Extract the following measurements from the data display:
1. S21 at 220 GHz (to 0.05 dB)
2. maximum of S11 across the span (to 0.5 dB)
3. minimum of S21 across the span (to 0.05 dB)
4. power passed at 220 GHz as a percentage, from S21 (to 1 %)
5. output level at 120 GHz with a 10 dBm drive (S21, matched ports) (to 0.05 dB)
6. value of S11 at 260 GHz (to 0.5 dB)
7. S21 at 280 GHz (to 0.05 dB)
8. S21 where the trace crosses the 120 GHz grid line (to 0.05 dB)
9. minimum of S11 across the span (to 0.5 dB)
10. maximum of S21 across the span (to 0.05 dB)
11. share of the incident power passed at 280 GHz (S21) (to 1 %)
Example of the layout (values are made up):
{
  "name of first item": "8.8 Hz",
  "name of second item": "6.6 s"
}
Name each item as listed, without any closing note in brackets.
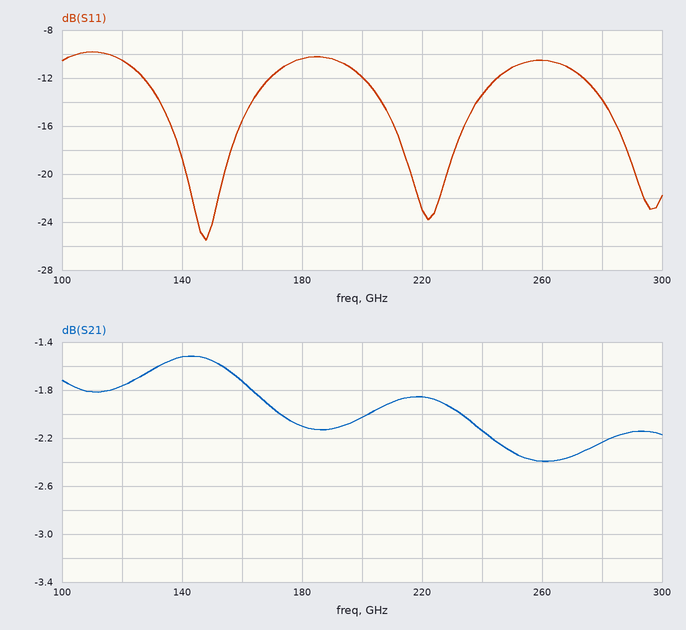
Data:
{
  "S21 at 220 GHz": "-1.85 dB",
  "maximum of S11 across the span": "-10.0 dB",
  "minimum of S21 across the span": "-2.40 dB",
  "power passed at 220 GHz as a percentage, from S21": "65 %",
  "output level at 120 GHz with a 10 dBm drive (S21, matched ports)": "8.25 dBm",
  "value of S11 at 260 GHz": "-10.5 dB",
  "S21 at 280 GHz": "-2.25 dB",
  "S21 where the trace crosses the 120 GHz grid line": "-1.75 dB",
  "minimum of S11 across the span": "-25.5 dB",
  "maximum of S21 across the span": "-1.50 dB",
  "share of the incident power passed at 280 GHz (S21)": "60 %"
}
